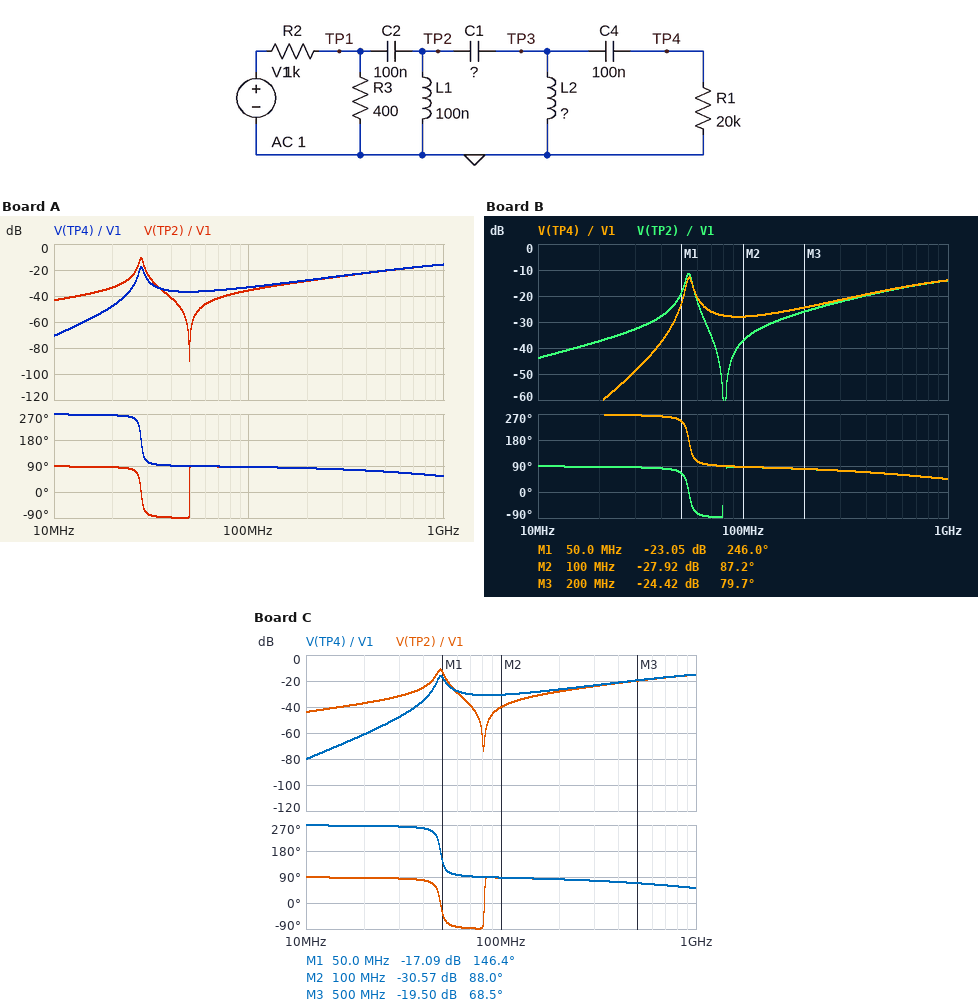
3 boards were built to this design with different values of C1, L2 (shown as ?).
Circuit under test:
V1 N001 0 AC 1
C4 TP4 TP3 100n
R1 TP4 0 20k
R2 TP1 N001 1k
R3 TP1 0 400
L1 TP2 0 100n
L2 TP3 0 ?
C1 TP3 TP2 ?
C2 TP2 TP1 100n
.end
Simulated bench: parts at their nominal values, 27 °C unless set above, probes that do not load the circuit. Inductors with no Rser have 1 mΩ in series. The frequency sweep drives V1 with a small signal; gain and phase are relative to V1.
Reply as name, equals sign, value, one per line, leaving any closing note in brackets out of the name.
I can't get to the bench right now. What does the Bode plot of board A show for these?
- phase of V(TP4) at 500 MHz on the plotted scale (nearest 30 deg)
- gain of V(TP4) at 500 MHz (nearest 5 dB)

phase of V(TP4) at 500 MHz on the plotted scale = 60 deg
gain of V(TP4) at 500 MHz = -20 dB
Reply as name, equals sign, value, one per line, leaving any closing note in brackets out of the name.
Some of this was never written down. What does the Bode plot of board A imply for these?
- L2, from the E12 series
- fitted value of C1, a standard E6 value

L2, from the E12 series = 47 nH
fitted value of C1, a standard E6 value = 220 pF
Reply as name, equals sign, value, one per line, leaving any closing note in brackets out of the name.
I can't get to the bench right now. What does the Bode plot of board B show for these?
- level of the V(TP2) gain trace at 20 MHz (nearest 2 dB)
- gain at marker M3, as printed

level of the V(TP2) gain trace at 20 MHz = -38 dB
gain at marker M3, as printed = -24.42 dB
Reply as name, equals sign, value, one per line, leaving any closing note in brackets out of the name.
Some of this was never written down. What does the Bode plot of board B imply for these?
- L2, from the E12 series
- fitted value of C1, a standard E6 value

L2, from the E12 series = 82 nH
fitted value of C1, a standard E6 value = 47 pF
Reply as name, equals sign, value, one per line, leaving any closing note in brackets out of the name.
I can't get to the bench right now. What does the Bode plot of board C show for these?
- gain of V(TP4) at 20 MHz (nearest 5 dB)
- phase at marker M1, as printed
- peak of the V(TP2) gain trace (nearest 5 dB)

gain of V(TP4) at 20 MHz = -60 dB
phase at marker M1, as printed = 146.4 deg
peak of the V(TP2) gain trace = -10 dB
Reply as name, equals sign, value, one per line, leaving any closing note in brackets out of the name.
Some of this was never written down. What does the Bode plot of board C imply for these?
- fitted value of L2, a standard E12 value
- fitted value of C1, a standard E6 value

fitted value of L2, a standard E12 value = 56 nH
fitted value of C1, a standard E6 value = 68 pF
